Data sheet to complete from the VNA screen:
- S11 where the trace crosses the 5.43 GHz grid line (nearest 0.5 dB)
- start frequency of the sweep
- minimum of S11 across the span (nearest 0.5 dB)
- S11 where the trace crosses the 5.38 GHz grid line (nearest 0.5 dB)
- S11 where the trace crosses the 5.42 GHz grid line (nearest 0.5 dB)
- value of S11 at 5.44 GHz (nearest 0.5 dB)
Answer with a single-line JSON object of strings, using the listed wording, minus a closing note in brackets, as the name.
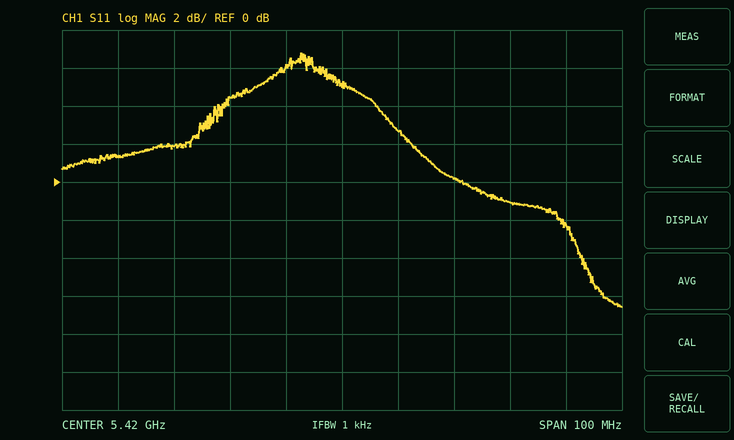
{"S11 where the trace crosses the 5.43 GHz grid line": "2.5 dB", "start frequency of the sweep": "5.37 GHz", "minimum of S11 across the span": "-6.5 dB", "S11 where the trace crosses the 5.38 GHz grid line": "1.5 dB", "S11 where the trace crosses the 5.42 GHz grid line": "5.0 dB", "value of S11 at 5.44 GHz": "0.0 dB"}
